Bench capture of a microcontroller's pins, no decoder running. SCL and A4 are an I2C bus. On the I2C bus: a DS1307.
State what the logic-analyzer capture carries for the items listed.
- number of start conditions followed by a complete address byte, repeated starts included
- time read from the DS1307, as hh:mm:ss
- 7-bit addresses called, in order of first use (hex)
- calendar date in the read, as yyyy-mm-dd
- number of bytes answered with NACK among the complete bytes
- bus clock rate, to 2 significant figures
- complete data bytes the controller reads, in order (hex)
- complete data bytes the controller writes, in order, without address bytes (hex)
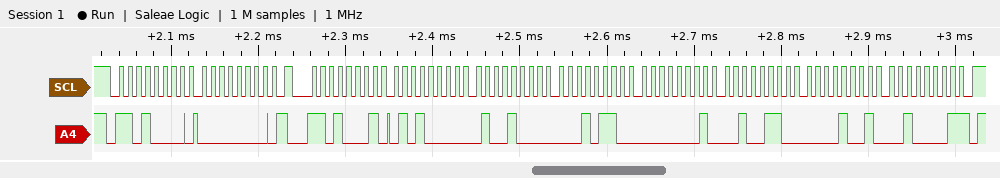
2
16:48:50
0x68
2021-09-26
1
100 kHz
50 48 16 01 26 09 21
00
